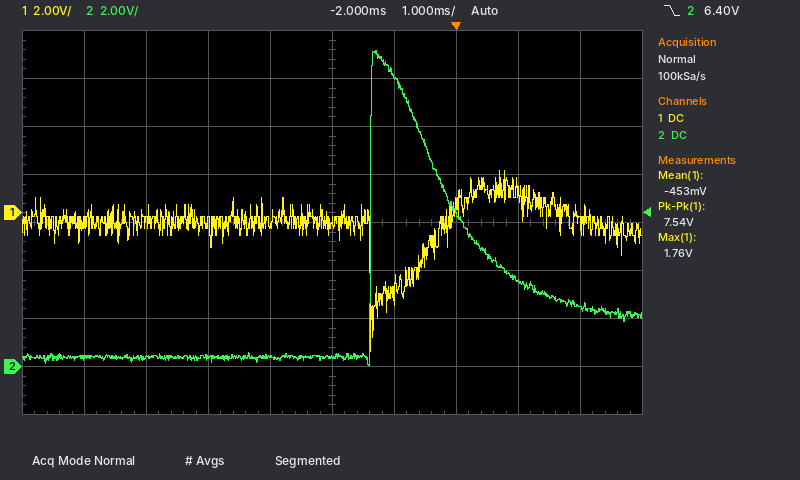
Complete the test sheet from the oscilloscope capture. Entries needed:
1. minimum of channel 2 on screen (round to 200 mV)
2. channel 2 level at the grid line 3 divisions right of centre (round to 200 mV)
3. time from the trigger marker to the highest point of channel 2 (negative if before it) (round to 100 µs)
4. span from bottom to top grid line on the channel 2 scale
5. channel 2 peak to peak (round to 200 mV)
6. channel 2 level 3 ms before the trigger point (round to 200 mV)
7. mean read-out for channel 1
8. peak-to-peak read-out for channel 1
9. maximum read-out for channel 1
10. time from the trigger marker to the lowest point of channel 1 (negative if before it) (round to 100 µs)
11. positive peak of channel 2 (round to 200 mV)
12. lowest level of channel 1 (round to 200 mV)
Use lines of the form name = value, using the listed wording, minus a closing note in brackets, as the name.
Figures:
minimum of channel 2 on screen = 0.0 V
channel 2 level at the grid line 3 divisions right of centre = 3.6 V
time from the trigger marker to the highest point of channel 2 (negative if before it) = -1.3 ms
span from bottom to top grid line on the channel 2 scale = 16 V
channel 2 peak to peak = 13.2 V
channel 2 level 3 ms before the trigger point = 400 mV
mean read-out for channel 1 = -453 mV
peak-to-peak read-out for channel 1 = 7.54 V
maximum read-out for channel 1 = 1.76 V
time from the trigger marker to the lowest point of channel 1 (negative if before it) = -1.4 ms
positive peak of channel 2 = 13.2 V
lowest level of channel 1 = -5.8 V
